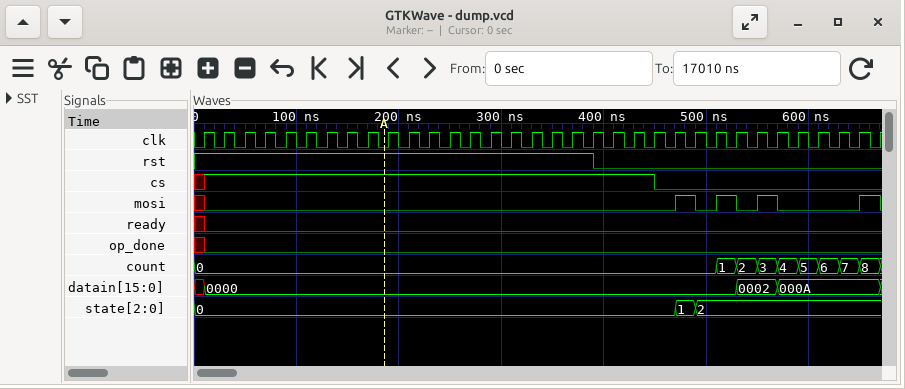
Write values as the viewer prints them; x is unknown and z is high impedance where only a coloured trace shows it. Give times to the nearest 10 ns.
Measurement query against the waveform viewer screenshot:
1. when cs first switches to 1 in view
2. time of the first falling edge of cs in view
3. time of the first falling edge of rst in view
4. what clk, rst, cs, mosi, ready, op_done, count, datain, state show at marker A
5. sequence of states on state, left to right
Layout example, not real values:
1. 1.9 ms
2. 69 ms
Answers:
1. 10 ns
2. 450 ns
3. 390 ns
4. clk=0, rst=1, cs=1, mosi=0, ready=0, op_done=0, count=0, datain=0000, state=0
5. 0, 1, 2
